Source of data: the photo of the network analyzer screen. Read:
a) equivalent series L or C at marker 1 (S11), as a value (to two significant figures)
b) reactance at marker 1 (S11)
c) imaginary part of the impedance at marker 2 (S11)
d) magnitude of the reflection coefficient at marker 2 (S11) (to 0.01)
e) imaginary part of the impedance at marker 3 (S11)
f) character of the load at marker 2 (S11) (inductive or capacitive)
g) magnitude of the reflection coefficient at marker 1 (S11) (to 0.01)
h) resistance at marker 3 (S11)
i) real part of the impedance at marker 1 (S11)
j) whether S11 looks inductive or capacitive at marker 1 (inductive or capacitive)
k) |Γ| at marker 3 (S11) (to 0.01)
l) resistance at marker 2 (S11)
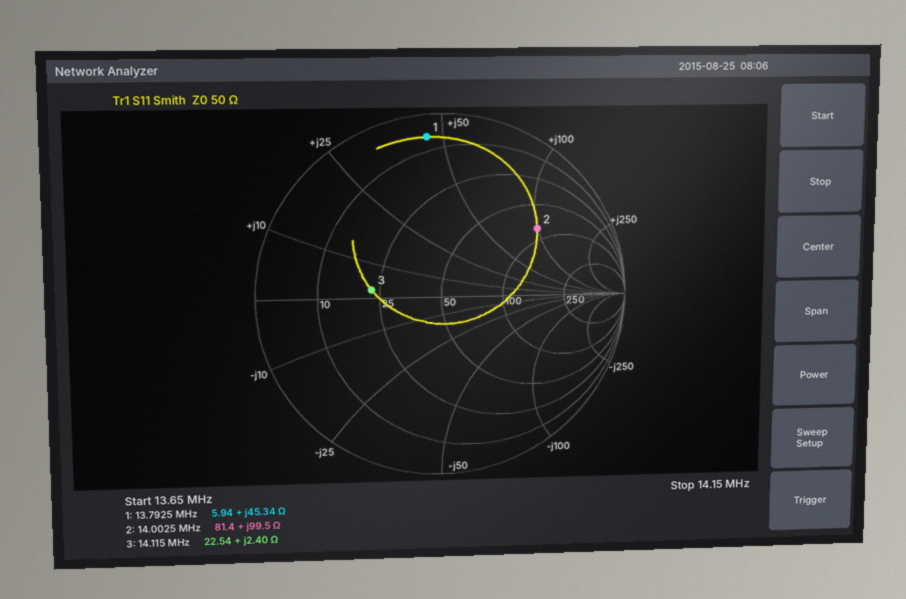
520 nH
+45.34 Ω
+99.5 Ω
0.63
+2.40 Ω
inductive
0.88
22.54 Ω
5.94 Ω
inductive
0.38
81.4 Ω
